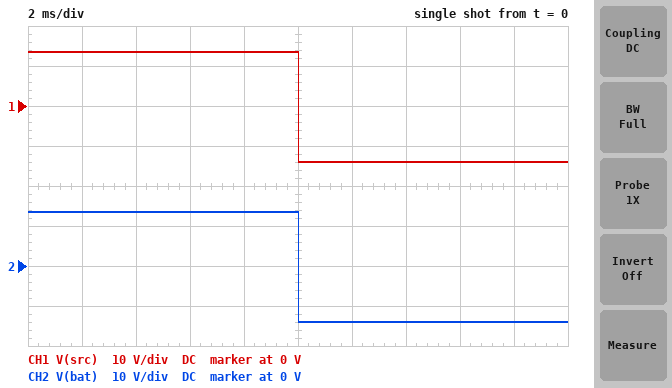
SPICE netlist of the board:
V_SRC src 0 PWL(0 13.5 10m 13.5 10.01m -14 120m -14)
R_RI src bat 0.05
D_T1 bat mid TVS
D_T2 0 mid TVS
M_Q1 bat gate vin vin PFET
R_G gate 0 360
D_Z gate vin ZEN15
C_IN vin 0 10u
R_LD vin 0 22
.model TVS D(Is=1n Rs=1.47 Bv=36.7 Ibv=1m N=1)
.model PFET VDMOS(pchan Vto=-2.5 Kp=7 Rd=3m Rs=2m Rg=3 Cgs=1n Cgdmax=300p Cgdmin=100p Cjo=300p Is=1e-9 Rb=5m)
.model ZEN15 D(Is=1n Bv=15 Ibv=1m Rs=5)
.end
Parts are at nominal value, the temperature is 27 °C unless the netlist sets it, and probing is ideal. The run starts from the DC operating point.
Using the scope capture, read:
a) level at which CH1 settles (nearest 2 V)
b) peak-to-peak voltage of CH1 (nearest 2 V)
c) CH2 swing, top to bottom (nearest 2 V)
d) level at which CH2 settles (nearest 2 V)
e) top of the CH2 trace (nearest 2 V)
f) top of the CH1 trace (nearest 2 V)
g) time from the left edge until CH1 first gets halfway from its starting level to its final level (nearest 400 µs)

-14 V
28 V
28 V
-14 V
14 V
14 V
10.0 ms
